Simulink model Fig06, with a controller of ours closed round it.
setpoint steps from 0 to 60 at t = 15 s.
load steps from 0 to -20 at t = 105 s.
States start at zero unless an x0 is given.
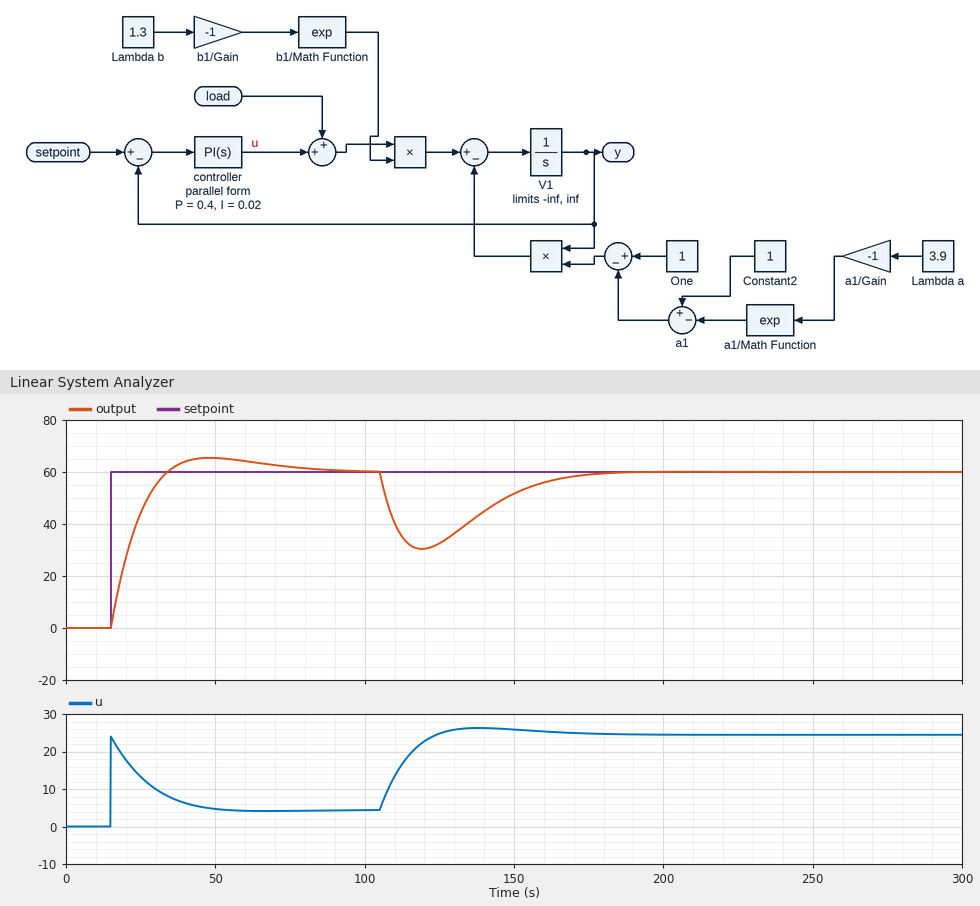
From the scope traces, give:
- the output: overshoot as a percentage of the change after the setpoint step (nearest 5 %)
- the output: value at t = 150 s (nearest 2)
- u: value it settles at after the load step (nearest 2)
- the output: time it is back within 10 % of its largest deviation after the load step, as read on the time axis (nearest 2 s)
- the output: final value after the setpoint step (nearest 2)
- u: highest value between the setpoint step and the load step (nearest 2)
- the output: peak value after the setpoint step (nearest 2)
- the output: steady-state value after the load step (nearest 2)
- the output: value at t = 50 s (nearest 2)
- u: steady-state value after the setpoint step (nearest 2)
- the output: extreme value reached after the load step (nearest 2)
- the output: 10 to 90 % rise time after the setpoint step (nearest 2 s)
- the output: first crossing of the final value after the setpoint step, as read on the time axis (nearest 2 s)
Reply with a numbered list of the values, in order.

1. 10 %
2. 52
3. 24
4. 164 s
5. 60
6. 24
7. 66
8. 60
9. 66
10. 4
11. 30
12. 14 s
13. 34 s
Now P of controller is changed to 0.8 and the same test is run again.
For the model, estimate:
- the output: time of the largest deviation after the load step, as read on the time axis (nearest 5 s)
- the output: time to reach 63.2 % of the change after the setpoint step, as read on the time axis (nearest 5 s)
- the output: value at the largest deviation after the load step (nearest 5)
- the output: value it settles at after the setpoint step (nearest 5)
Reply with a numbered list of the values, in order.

1. 115 s
2. 20 s
3. 40
4. 60
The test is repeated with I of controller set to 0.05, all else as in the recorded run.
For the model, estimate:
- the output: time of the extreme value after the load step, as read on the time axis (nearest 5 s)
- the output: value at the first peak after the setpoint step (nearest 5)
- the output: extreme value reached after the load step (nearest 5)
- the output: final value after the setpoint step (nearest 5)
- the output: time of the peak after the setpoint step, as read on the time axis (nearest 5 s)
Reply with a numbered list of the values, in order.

1. 115 s
2. 75
3. 35
4. 60
5. 35 s
